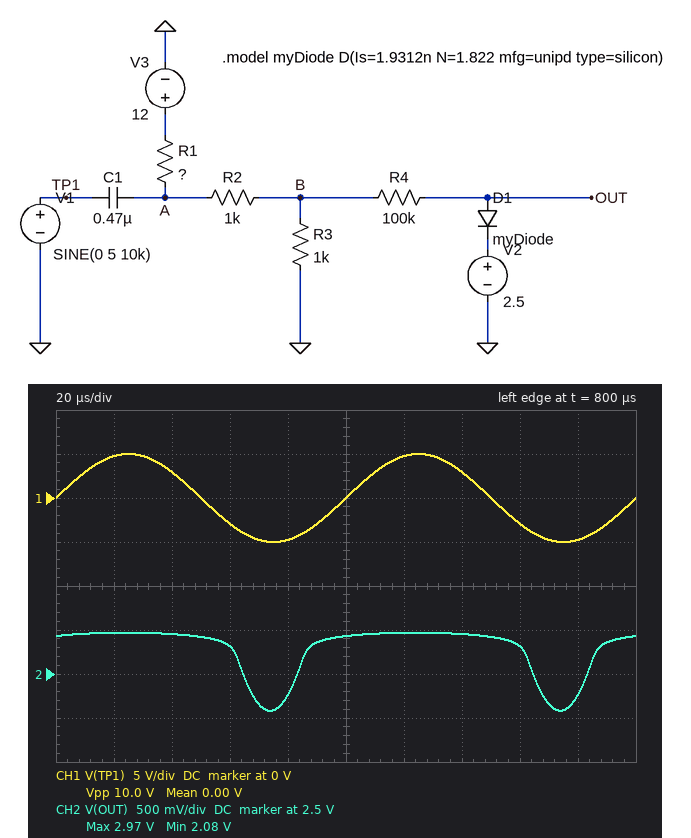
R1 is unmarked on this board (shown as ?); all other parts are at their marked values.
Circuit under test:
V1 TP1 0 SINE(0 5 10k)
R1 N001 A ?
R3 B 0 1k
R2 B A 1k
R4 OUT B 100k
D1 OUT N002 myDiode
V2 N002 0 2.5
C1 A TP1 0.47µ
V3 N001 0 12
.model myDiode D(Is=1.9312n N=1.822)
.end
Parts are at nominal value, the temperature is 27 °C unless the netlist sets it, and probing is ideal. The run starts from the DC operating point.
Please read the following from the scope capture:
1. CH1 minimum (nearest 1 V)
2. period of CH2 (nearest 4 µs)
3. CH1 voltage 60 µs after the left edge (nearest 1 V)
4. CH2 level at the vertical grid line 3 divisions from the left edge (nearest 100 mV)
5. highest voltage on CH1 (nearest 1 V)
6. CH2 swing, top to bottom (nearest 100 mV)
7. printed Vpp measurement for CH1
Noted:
-5 V
100 µs
-3 V
2.8 V
5 V
900 mV
10.0 V
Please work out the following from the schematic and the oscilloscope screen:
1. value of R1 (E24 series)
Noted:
620 Ω
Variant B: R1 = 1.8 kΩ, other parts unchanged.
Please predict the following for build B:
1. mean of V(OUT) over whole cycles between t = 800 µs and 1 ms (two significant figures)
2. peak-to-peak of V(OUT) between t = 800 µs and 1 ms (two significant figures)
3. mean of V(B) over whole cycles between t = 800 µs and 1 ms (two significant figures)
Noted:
2.2 V
2.3 V
3.1 V
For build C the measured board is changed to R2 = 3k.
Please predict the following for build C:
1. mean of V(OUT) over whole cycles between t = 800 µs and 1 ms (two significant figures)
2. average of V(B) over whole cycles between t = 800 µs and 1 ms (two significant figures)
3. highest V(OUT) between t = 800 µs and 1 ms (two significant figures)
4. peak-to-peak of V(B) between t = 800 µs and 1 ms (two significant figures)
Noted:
2.3 V
2.6 V
2.9 V
2.5 V
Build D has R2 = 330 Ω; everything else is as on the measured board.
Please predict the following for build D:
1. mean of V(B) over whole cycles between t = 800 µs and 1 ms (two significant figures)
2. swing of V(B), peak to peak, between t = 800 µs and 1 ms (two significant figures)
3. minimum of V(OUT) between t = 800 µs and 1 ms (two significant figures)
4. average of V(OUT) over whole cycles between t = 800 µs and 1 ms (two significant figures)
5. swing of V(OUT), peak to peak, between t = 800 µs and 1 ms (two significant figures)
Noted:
6.1 V
7.5 V
2.4 V
2.9 V
600 mV
